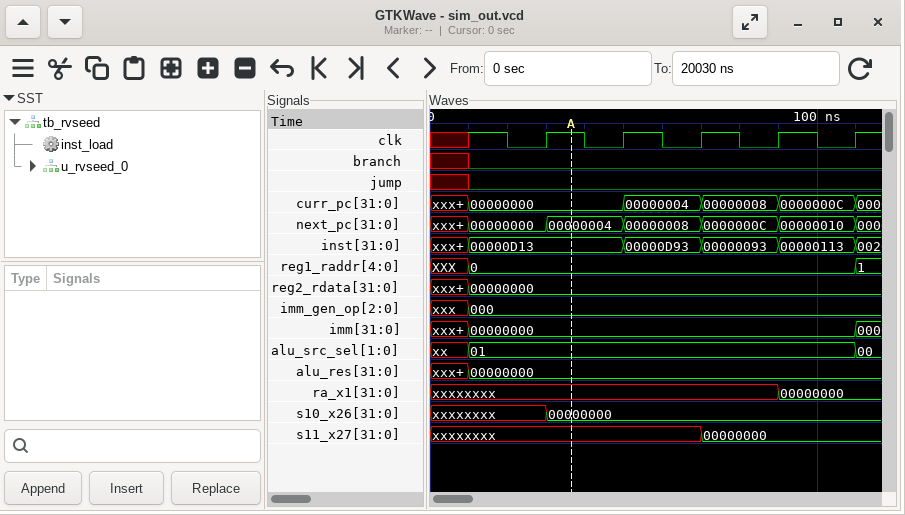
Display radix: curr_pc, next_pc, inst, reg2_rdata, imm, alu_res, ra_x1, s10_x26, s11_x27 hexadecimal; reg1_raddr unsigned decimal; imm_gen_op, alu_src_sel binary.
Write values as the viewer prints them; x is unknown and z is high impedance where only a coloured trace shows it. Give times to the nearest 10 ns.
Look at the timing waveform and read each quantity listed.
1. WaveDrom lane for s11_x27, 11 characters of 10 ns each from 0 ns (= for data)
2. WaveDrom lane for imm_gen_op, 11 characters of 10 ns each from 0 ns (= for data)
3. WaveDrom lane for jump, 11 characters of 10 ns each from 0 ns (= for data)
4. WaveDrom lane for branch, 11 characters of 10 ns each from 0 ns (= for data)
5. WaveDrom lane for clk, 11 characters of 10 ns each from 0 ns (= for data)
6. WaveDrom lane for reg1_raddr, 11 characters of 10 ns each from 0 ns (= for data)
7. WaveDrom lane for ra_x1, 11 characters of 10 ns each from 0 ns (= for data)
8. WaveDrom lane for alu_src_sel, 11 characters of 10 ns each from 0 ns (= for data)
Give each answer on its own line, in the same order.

{name: 's11_x27', wave: 'x......=...', data: '00000000'}
{name: 'imm_gen_op', wave: 'x=.........', data: '000'}
{name: 'jump', wave: 'x0.........'}
{name: 'branch', wave: 'x0.........'}
{name: 'clk', wave: 'x1010101010'}
{name: 'reg1_raddr', wave: 'x=.........', data: '0'}
{name: 'ra_x1', wave: 'x........=.', data: '00000000'}
{name: 'alu_src_sel', wave: 'x=.........', data: '01'}
